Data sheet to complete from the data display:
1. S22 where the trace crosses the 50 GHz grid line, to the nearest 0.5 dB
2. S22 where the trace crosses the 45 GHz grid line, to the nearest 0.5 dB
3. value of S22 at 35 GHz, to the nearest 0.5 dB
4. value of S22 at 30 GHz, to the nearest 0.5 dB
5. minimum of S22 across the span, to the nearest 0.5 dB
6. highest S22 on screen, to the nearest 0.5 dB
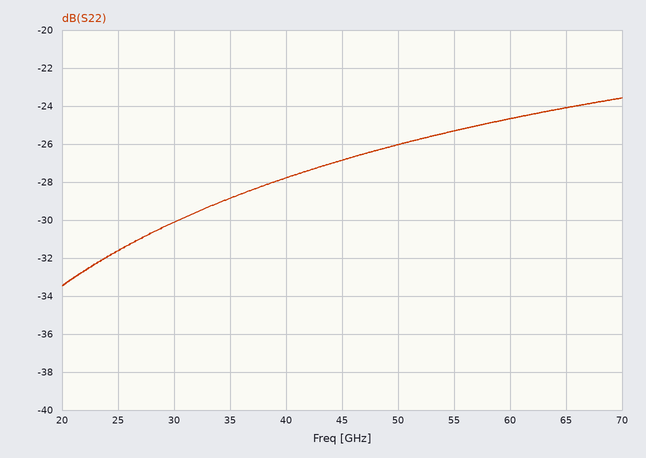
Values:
-26.0 dB
-27.0 dB
-29.0 dB
-30.0 dB
-33.5 dB
-23.5 dB
